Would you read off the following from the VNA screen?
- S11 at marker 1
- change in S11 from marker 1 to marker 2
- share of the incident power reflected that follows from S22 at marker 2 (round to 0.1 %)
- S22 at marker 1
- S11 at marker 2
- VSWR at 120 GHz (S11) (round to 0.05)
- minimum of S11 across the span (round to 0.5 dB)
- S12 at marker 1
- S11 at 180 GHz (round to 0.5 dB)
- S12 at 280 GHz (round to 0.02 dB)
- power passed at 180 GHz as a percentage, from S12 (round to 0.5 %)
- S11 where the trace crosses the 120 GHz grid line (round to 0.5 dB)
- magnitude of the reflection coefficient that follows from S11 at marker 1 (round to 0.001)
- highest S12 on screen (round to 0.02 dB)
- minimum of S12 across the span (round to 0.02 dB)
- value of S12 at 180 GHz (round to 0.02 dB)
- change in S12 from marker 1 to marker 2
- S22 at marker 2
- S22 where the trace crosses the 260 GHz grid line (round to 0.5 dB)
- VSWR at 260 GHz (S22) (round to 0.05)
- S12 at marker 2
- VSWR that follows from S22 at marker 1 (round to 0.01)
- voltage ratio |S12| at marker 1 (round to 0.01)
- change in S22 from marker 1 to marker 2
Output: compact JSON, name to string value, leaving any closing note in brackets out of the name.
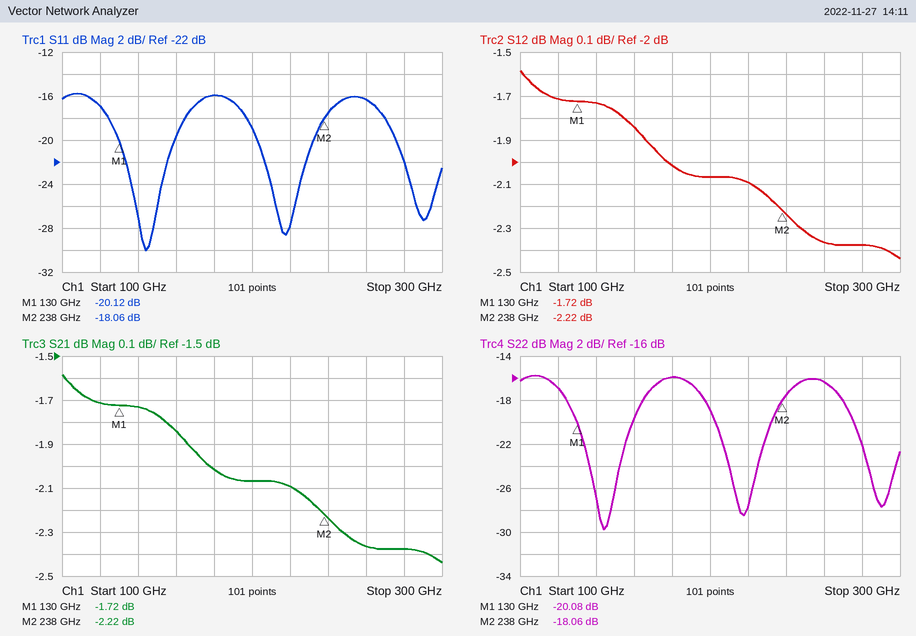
{"S11 at marker 1": "-20.12 dB", "change in S11 from marker 1 to marker 2": "2.06 dB", "share of the incident power reflected that follows from S22 at marker 2": "1.6 %", "S22 at marker 1": "-20.08 dB", "S11 at marker 2": "-18.06 dB", "VSWR at 120 GHz (S11)": "1.35", "minimum of S11 across the span": "-30.0 dB", "S12 at marker 1": "-1.72 dB", "S11 at 180 GHz": "-16.0 dB", "S12 at 280 GHz": "-2.38 dB", "power passed at 180 GHz as a percentage, from S12": "63.0 %", "S11 where the trace crosses the 120 GHz grid line": "-17.0 dB", "magnitude of the reflection coefficient that follows from S11 at marker 1": "0.099", "highest S12 on screen": "-1.58 dB", "minimum of S12 across the span": "-2.44 dB", "value of S12 at 180 GHz": "-2.02 dB", "change in S12 from marker 1 to marker 2": "-0.50 dB", "S22 at marker 2": "-18.06 dB", "S22 where the trace crosses the 260 GHz grid line": "-16.5 dB", "VSWR at 260 GHz (S22)": "1.35", "S12 at marker 2": "-2.22 dB", "VSWR that follows from S22 at marker 1": "1.22", "voltage ratio |S12| at marker 1": "0.82", "change in S22 from marker 1 to marker 2": "2.02 dB"}
